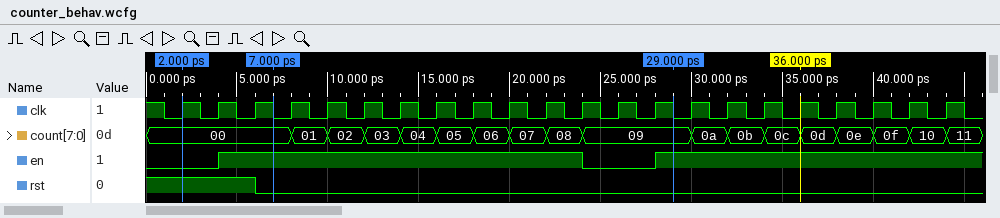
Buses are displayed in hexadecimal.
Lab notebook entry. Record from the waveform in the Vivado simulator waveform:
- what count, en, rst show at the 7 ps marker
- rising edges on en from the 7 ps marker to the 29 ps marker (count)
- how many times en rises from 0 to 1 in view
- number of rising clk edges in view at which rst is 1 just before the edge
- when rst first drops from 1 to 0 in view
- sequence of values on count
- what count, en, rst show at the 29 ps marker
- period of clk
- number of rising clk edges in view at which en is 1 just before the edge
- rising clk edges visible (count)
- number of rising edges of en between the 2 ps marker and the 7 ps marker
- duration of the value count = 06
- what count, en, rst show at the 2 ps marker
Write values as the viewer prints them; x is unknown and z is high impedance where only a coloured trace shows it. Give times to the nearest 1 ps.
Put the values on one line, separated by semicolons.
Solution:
count=00, en=1, rst=0; 1; 2; 3; 6 ps; 00, 01, 02, 03, 04, 05, 06, 07, 08, 09, 0a, 0b, 0c, 0d, 0e, 0f, 10, 11; count=09, en=1, rst=0; 2 ps; 18; 22; 1; 2 ps; count=00, en=0, rst=1
